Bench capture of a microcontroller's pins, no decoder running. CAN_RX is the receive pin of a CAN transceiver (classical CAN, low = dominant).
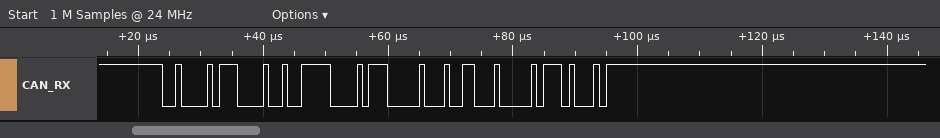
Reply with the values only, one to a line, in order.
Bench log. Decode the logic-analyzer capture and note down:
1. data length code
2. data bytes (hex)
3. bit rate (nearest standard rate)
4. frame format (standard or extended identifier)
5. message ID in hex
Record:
4
9F 17 00 98
1000 kbit/s
standard
0x217
